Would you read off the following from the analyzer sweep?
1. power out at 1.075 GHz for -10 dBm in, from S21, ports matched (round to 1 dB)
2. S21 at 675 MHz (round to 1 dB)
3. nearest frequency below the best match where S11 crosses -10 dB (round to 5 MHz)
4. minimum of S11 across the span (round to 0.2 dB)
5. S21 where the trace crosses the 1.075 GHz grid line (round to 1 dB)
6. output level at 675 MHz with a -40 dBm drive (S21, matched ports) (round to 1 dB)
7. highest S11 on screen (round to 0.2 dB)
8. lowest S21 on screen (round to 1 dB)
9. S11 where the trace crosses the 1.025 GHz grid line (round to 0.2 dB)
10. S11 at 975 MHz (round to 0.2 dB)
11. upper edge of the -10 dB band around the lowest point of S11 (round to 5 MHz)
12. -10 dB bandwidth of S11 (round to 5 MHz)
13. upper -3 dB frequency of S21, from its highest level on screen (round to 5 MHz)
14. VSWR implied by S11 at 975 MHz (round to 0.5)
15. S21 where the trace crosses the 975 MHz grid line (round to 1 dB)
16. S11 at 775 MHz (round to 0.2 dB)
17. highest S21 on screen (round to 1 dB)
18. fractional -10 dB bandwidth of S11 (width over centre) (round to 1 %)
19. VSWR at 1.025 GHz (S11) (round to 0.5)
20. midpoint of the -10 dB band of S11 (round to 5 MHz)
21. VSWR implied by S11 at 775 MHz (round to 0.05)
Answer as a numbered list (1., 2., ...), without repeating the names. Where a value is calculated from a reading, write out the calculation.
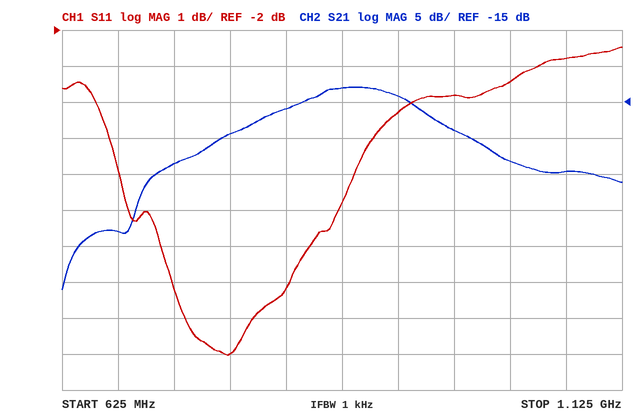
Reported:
1. -10 dBm + (-25 dB) = -35 dBm
2. -33 dB
3. 735 MHz
4. -11.0 dB
5. -25 dB
6. -40 dBm + (-33 dB) = -73 dBm
7. -2.4 dB
8. -41 dB
9. -3.4 dB
10. -3.8 dB
11. 795 MHz
12. 795 MHz − 735 MHz = 60 MHz
13. 945 MHz
14. |Γ| = 10^(-3.8/20) = 0.6457; VSWR = (1 + 0.6457)/(1 − 0.6457) ≈ 4.64, so 4.5 to the nearest 0.5
15. -19 dB
16. -11.0 dB
17. -13 dB
18. 60 MHz / 765 MHz ≈ 8 %
19. |Γ| = 10^(-3.4/20) = 0.6761; VSWR = (1 + 0.6761)/(1 − 0.6761) ≈ 5.17, so 5.0 to the nearest 0.5
20. 765 MHz
21. |Γ| = 10^(-11/20) = 0.2818; VSWR = (1 + 0.2818)/(1 − 0.2818) ≈ 1.78, so 1.80 to the nearest 0.05
